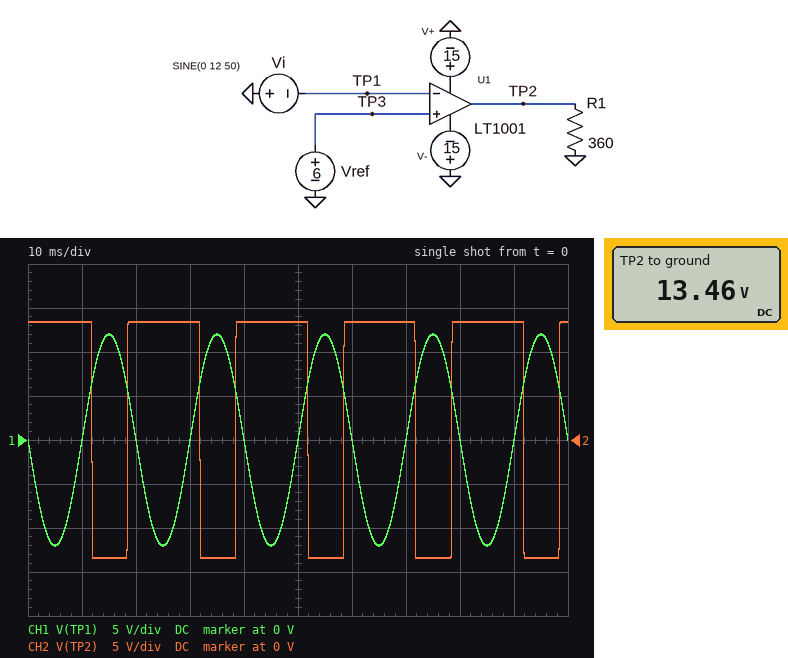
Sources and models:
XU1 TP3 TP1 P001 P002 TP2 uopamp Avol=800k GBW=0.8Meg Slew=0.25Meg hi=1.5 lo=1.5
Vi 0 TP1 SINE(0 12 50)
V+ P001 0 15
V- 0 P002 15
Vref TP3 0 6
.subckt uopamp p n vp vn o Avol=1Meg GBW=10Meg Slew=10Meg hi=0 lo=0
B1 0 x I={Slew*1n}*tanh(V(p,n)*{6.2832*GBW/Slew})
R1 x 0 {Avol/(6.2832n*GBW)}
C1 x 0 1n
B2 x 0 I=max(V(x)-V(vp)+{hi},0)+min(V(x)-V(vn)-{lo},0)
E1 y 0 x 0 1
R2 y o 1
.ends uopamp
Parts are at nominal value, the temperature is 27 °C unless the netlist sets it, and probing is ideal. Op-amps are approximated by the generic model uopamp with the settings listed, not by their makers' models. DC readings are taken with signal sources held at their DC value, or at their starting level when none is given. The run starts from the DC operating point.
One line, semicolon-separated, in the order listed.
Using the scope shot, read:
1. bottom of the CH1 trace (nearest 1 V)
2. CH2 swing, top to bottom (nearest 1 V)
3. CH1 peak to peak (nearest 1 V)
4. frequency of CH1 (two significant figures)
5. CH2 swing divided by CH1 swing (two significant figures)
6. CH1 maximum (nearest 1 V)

-12 V; 27 V; 24 V; 50 Hz; 1.1; 12 V
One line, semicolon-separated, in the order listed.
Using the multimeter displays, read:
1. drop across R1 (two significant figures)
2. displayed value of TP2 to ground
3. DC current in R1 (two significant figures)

13 V; 13.46 V; 37 mA
